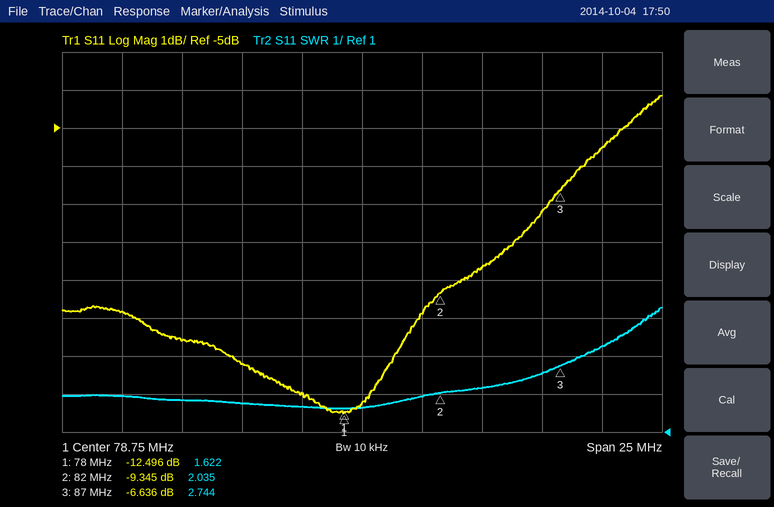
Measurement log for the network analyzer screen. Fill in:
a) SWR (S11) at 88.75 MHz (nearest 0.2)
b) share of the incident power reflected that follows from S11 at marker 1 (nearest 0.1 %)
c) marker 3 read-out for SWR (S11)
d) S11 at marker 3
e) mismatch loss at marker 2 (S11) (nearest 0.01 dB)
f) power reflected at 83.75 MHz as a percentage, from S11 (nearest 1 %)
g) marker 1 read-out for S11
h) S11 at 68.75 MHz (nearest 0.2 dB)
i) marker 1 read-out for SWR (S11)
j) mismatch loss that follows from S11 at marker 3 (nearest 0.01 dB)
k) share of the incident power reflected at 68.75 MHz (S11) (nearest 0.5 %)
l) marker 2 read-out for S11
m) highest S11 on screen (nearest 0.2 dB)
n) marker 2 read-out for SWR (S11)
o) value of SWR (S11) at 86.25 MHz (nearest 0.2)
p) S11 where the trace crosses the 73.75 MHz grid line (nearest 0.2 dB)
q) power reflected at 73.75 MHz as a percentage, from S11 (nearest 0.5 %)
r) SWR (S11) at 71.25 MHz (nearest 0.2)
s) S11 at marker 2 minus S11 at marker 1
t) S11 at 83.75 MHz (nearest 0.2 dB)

3.2
5.6 %
2.744
-6.636 dB
0.54 dB
14 %
-12.496 dB
-9.8 dB
1.622
1.06 dB
10.5 %
-9.345 dB
-4.2 dB
2.035
2.6
-11.2 dB
7.5 %
1.8
3.151 dB
-8.6 dB
